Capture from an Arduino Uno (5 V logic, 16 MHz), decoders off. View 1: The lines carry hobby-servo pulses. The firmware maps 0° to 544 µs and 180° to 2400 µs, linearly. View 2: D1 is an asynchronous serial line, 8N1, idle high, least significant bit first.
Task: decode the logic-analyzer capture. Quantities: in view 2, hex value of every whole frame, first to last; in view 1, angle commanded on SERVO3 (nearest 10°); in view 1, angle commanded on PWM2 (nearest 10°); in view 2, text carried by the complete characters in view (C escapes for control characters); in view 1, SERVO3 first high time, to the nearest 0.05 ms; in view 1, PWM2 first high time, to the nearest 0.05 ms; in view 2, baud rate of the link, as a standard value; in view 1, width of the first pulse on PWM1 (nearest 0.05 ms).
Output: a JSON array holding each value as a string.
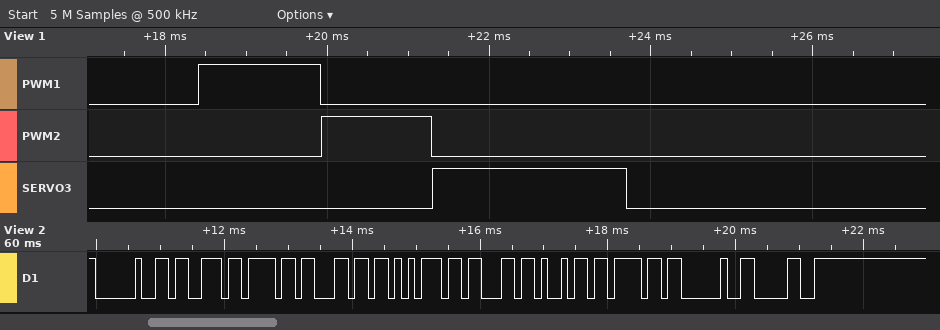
["0x20 0x73 0x6F 0x6C 0x75 0x63 0x69 0x6F 0x20 0x30", "180°", "80°", "\" solucio 0\"", "2.40 ms", "1.35 ms", "9600 baud", "1.50 ms"]
